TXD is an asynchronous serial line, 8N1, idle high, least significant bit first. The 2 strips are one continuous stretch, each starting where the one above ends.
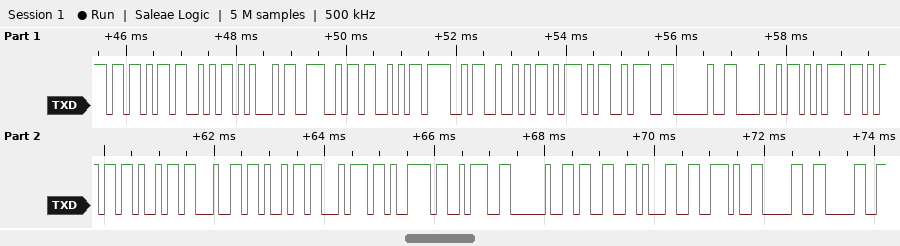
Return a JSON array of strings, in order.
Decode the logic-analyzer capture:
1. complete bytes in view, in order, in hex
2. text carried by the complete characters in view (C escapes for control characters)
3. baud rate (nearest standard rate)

["5B 53 45 4E 53 4F 52 5D 3A 20 48 75 6D 69 64 69 74 79 3A 20 33 31 2E 30 30", "\"[SENSOR]: Humidity: 31.00\"", "9600 baud"]
